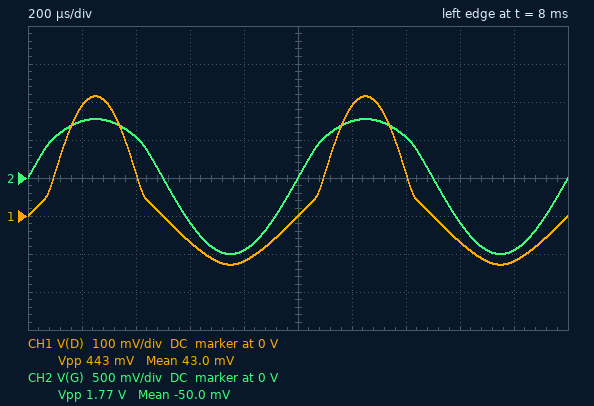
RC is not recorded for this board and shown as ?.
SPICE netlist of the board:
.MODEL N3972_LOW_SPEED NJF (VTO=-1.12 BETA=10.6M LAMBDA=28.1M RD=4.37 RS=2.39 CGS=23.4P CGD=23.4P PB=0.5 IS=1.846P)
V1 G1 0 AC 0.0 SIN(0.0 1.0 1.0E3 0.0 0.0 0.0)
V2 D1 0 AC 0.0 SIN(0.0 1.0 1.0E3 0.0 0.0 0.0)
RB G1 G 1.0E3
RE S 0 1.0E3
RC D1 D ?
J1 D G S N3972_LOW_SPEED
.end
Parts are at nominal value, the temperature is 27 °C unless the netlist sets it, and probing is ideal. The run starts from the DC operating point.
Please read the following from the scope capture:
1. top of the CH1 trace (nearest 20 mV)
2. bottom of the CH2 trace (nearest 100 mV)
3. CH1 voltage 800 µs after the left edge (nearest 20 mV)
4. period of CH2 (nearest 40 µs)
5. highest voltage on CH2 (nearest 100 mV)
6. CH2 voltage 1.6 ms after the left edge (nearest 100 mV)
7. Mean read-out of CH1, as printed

320 mV
-1.0 V
-120 mV
1.00 ms
800 mV
-600 mV
43.0 mV
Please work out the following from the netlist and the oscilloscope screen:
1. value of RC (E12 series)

8.2 kΩ
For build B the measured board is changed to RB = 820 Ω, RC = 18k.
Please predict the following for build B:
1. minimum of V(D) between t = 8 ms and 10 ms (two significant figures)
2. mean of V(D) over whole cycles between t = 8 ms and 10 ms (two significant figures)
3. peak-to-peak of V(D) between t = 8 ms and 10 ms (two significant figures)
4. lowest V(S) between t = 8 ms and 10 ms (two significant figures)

-66 mV
58 mV
380 mV
-52 mV
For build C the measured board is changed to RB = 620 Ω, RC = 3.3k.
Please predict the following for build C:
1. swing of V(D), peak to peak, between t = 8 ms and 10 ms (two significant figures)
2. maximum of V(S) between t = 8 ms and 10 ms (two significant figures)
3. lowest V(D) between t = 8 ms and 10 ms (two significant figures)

660 mV
400 mV
-260 mV
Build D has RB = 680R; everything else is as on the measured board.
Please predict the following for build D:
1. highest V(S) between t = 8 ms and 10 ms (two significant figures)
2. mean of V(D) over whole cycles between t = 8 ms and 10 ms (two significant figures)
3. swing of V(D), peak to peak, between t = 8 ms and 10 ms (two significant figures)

350 mV
51 mV
480 mV
